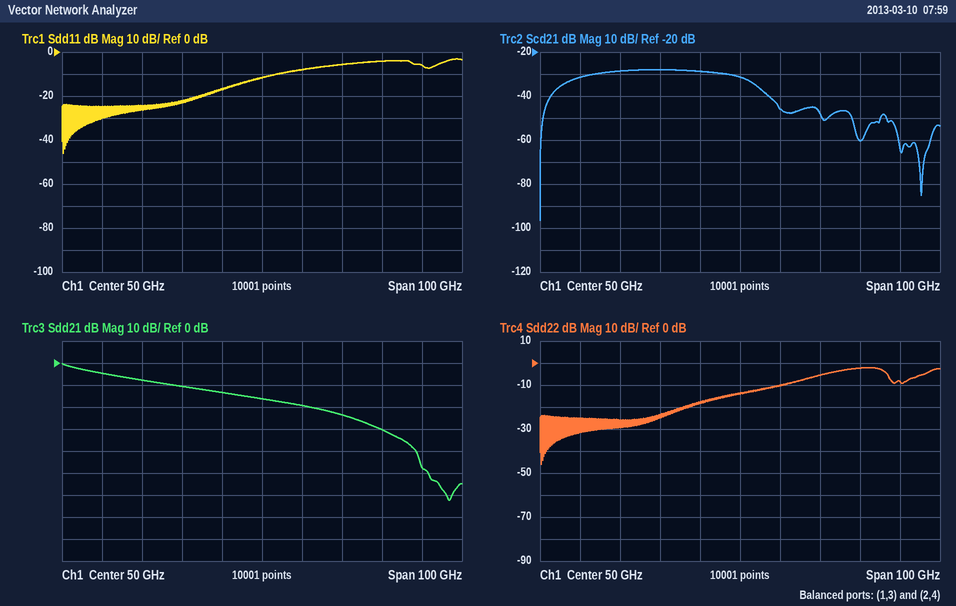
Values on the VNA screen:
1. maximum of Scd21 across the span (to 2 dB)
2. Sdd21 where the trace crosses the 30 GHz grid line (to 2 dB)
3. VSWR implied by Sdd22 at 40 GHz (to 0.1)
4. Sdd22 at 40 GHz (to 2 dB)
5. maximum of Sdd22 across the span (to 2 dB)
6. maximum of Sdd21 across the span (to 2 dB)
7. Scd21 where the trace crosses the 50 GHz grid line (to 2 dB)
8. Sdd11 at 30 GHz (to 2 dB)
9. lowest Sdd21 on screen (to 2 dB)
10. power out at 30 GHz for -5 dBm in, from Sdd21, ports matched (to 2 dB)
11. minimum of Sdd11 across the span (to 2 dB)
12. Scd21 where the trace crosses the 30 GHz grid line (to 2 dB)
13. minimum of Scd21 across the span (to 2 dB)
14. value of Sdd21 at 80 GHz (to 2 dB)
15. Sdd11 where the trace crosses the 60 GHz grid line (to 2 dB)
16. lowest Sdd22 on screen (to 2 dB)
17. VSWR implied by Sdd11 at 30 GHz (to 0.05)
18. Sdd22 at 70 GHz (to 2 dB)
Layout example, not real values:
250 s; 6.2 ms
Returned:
-28 dB; -10 dB; 1.3; -18 dB; -2 dB; 0 dB; -32 dB; -22 dB; -62 dB; -16 dBm; -46 dB; -28 dB; -96 dB; -30 dB; -8 dB; -46 dB; 1.15; -6 dB
